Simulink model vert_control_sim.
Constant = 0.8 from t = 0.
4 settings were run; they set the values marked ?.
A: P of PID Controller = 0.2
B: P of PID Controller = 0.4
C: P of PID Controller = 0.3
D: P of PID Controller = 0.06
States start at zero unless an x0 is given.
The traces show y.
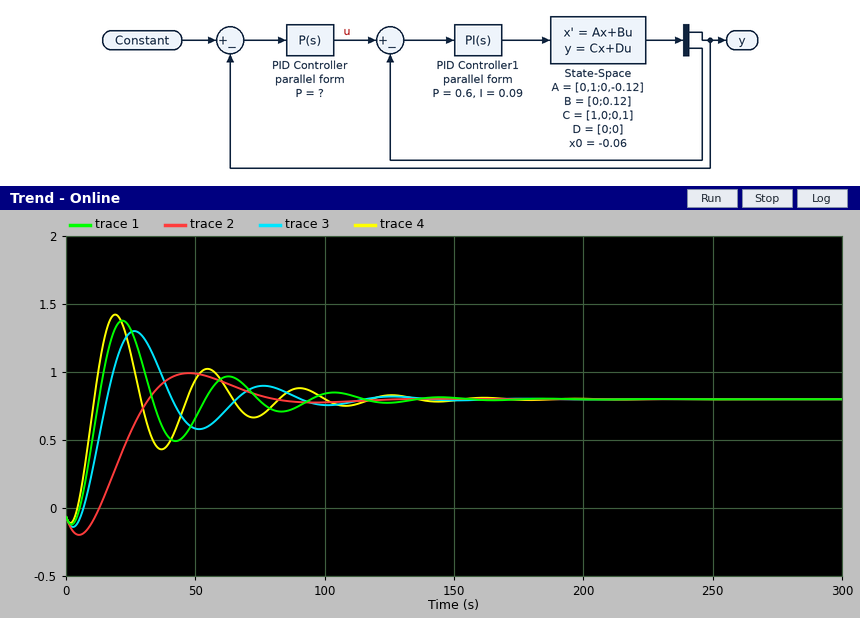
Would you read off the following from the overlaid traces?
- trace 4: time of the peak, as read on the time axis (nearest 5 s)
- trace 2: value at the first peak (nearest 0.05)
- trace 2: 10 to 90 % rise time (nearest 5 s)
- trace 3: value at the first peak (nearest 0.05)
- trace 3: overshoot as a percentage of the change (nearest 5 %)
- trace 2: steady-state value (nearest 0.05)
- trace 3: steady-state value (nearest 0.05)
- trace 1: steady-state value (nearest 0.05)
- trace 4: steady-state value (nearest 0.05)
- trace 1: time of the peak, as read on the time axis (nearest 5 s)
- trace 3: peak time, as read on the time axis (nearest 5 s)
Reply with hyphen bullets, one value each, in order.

- 20 s
- 1.00
- 15 s
- 1.30
- 60 %
- 0.80
- 0.80
- 0.80
- 0.80
- 20 s
- 25 s
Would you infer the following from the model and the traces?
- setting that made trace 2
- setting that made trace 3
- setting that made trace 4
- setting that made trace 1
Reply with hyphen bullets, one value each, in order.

- D
- A
- B
- C
